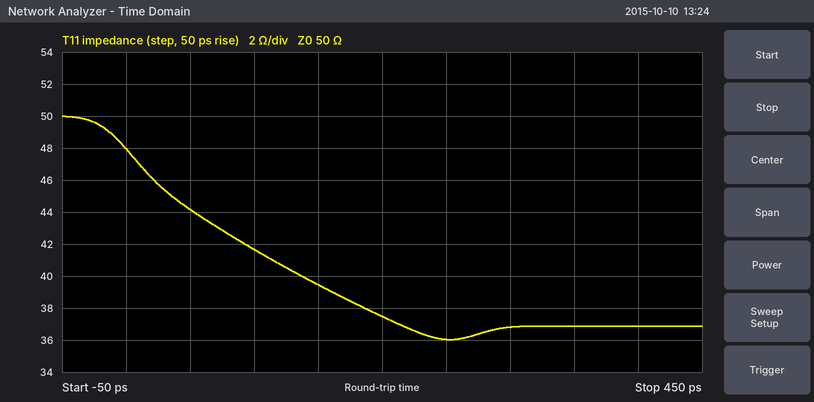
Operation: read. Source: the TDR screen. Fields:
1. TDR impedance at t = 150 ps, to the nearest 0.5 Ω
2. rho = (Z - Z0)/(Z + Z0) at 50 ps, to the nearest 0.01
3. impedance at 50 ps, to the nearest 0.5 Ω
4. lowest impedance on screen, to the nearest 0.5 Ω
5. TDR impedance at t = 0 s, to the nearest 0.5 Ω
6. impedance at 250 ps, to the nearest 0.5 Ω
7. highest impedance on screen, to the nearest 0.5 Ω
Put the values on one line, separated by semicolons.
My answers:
39.5 Ω; -0.06; 44.0 Ω; 36.0 Ω; 48.0 Ω; 36.0 Ω; 50.0 Ω
